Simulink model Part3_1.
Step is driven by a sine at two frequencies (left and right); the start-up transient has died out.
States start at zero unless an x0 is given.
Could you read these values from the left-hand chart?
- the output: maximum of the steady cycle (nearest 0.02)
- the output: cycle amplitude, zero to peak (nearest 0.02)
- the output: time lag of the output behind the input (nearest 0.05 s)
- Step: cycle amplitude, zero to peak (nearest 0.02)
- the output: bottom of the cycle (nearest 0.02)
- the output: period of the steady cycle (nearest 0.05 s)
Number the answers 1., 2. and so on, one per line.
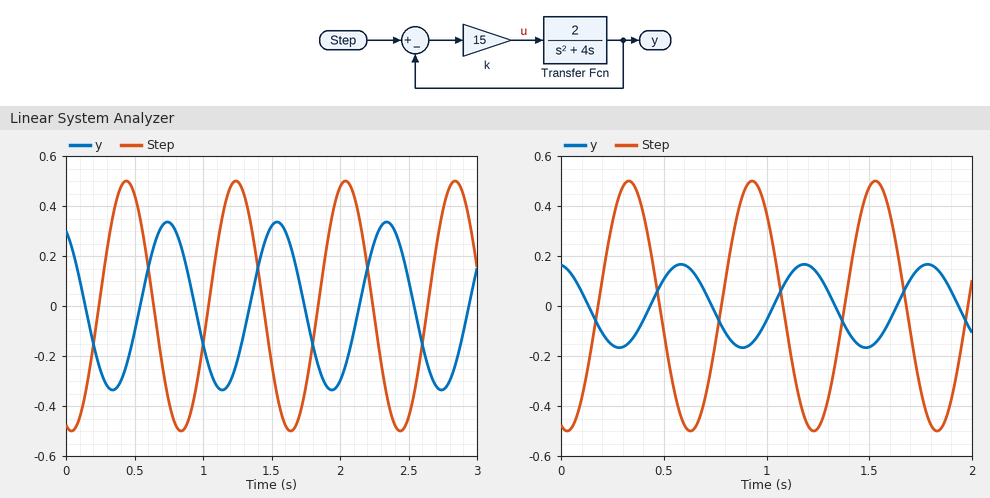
1. 0.34
2. 0.34
3. 0.30 s
4. 0.50
5. -0.34
6. 0.80 s
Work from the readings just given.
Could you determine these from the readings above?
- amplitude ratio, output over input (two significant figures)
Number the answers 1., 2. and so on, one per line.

1. 0.68
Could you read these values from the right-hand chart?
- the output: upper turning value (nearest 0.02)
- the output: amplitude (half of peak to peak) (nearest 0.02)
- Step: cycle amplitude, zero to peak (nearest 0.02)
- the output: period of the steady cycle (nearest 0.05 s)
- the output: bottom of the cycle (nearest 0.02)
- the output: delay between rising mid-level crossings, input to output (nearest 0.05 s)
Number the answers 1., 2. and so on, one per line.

1. 0.16
2. 0.16
3. 0.50
4. 0.60 s
5. -0.16
6. 0.25 s
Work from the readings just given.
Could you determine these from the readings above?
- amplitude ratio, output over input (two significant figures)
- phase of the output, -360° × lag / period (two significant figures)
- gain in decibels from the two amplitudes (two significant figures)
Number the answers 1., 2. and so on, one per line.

1. 0.32
2. -150°
3. -9.9 dB
